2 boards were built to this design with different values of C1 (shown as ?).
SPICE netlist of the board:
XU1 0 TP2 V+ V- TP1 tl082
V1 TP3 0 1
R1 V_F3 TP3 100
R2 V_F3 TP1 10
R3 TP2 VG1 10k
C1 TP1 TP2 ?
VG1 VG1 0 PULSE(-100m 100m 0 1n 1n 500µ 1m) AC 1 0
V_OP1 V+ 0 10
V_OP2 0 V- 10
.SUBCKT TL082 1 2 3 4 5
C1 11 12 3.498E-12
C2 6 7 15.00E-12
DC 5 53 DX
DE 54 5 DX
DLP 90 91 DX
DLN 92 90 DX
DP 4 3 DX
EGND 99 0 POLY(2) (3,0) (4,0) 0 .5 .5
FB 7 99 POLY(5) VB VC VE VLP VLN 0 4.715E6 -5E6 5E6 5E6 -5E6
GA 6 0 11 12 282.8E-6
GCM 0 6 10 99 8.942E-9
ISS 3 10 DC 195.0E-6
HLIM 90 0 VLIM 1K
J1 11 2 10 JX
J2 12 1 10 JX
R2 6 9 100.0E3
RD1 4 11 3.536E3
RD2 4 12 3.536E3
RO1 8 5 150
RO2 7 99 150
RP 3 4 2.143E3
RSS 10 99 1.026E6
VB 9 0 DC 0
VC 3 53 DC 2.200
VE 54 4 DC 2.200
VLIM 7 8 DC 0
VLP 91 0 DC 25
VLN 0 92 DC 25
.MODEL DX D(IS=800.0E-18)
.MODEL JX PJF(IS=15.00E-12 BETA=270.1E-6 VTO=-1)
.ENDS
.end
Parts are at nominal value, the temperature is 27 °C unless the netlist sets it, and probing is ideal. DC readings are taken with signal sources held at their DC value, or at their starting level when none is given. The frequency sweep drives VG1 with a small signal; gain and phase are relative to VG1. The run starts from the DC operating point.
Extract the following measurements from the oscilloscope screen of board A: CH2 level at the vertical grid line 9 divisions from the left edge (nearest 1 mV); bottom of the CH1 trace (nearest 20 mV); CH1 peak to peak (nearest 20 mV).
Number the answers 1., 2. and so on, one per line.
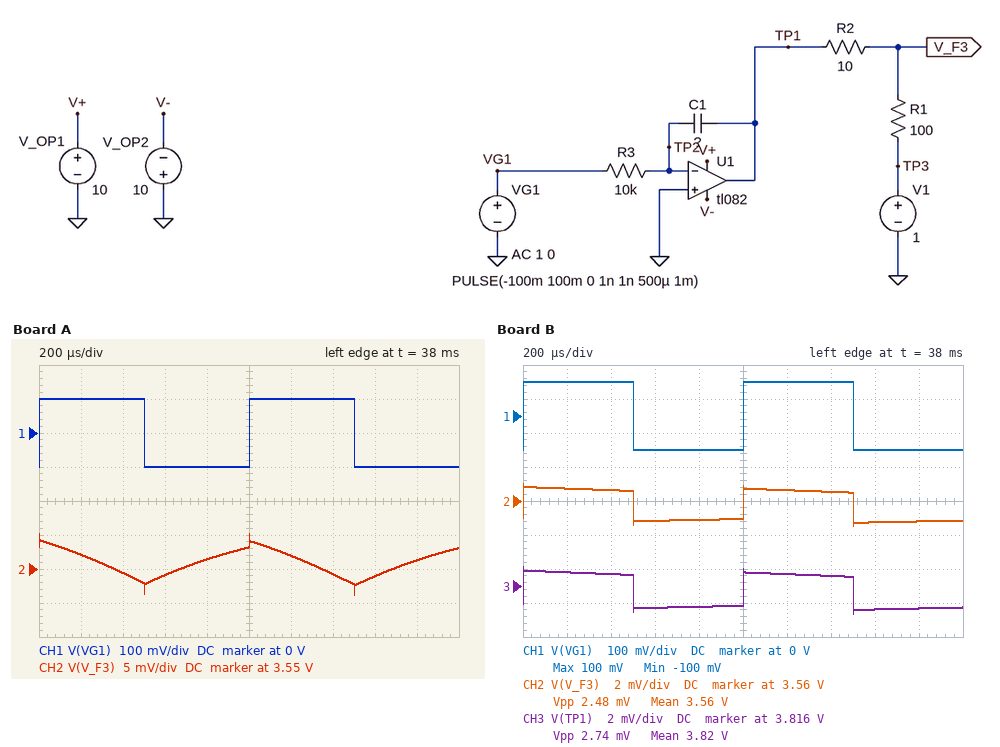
1. 3.551 V
2. -100 mV
3. 200 mV
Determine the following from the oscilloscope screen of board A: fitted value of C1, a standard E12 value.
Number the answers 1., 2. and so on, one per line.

1. 560 nF
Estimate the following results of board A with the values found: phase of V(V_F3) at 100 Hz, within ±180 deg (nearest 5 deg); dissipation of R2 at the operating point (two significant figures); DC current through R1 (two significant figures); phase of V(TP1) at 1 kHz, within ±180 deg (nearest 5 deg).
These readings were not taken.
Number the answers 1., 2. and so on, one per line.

1. 50 deg
2. 6.6 mW
3. 26 mA
4. 5 deg
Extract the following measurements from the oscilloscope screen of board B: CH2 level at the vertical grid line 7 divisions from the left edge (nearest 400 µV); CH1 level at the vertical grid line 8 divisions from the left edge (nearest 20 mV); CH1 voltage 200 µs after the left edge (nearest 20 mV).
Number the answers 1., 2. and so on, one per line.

1. 3.5604 V
2. -100 mV
3. 100 mV
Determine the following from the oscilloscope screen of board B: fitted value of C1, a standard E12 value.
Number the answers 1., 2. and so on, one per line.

1. 2.7 µF
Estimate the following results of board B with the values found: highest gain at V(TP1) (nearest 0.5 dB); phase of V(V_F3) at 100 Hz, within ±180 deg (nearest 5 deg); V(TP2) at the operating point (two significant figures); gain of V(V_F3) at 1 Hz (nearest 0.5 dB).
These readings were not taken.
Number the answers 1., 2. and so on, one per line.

1. -31.0 dB
2. 10 deg
3. -100 mV
4. -32.0 dB
